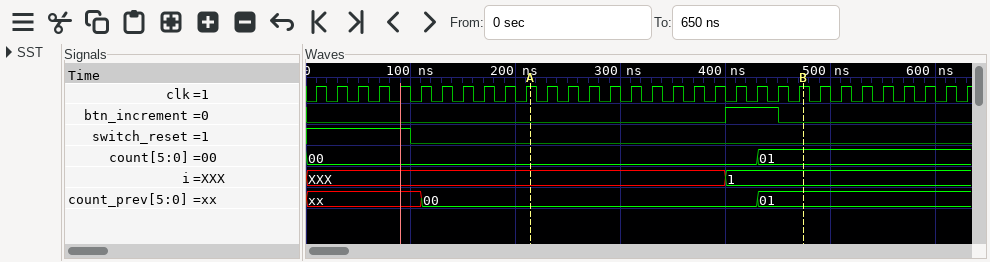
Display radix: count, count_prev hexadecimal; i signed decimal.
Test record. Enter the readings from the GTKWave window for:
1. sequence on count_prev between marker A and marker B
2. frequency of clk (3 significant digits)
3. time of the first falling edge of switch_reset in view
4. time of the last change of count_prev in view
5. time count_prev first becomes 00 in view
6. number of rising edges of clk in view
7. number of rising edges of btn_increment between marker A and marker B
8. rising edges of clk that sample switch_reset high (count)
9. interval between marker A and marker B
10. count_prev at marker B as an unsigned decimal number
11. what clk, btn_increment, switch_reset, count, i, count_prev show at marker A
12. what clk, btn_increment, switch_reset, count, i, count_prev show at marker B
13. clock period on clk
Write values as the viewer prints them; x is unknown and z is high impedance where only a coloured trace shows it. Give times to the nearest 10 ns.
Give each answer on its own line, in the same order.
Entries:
00, 01
50.0 MHz
100 ns
430 ns
110 ns
32
1
5
260 ns
1
clk=1, btn_increment=0, switch_reset=0, count=00, i=XXX, count_prev=00
clk=1, btn_increment=0, switch_reset=0, count=01, i=1, count_prev=01
20 ns
